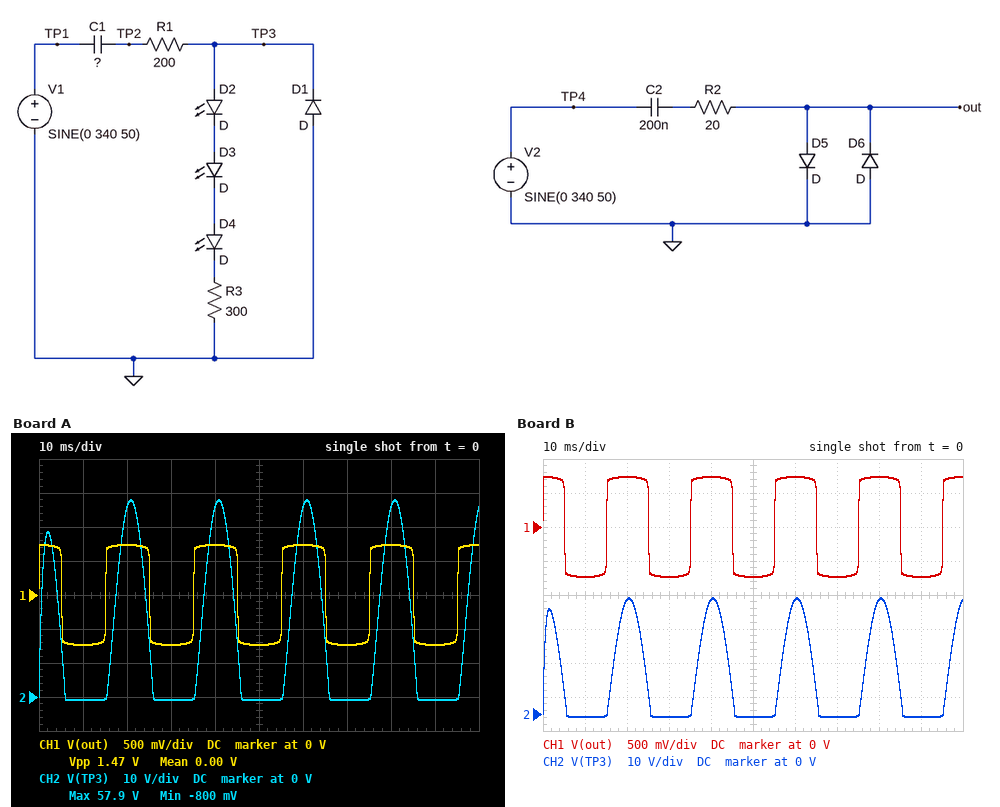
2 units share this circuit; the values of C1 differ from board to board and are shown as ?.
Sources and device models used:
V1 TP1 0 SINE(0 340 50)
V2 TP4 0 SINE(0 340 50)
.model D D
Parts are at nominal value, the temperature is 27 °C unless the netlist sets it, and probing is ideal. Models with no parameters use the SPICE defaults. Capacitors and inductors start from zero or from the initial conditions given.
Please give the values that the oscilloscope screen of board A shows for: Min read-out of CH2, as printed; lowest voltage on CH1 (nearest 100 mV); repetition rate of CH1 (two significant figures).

-800 mV
-700 mV
50 Hz
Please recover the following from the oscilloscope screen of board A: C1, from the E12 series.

1.8 µF
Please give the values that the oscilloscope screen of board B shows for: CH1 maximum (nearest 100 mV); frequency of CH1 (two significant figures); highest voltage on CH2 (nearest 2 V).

700 mV
50 Hz
34 V
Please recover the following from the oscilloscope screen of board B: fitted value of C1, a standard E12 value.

1 µF
